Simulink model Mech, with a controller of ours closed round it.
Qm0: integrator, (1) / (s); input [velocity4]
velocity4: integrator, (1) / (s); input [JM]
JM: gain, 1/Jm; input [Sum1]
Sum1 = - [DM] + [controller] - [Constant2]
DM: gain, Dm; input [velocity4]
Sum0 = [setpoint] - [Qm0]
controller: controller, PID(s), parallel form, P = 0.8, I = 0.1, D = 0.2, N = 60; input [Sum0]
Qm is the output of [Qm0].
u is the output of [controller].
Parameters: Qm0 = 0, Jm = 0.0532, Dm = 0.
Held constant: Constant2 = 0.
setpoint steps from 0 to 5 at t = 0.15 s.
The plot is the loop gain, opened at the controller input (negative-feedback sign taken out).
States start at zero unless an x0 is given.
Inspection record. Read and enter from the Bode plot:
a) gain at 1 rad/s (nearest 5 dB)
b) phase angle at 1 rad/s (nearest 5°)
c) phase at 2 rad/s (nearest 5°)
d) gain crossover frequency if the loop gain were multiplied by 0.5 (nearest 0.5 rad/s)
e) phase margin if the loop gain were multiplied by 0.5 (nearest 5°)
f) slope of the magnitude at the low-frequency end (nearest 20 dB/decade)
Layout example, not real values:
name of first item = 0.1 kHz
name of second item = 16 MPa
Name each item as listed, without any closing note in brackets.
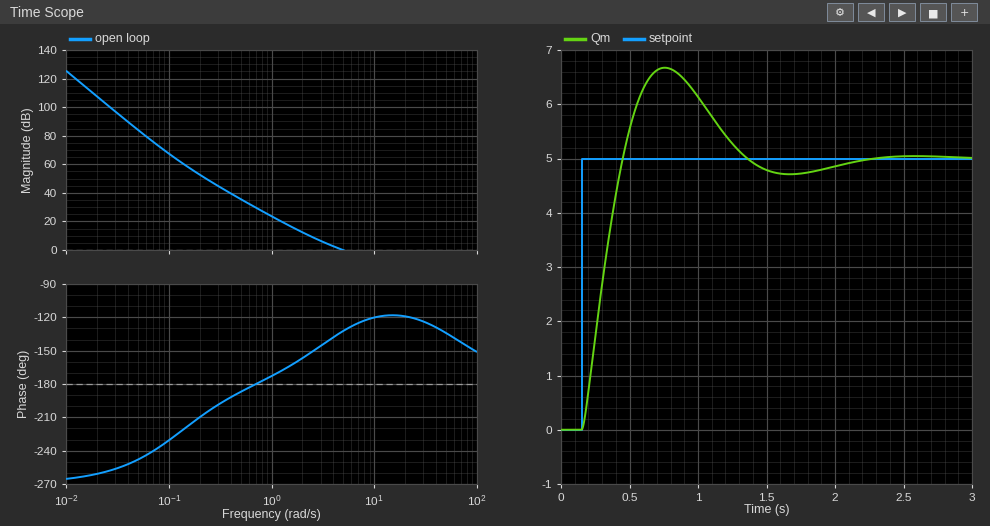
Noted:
gain at 1 rad/s = 25 dB
phase angle at 1 rad/s = -175°
phase at 2 rad/s = -155°
gain crossover frequency if the loop gain were multiplied by 0.5 = 3.0 rad/s
phase margin if the loop gain were multiplied by 0.5 = 35°
slope of the magnitude at the low-frequency end = -60 dB/decade
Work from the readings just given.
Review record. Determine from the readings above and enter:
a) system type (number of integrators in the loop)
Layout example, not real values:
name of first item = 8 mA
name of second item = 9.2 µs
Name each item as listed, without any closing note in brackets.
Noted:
system type = 3
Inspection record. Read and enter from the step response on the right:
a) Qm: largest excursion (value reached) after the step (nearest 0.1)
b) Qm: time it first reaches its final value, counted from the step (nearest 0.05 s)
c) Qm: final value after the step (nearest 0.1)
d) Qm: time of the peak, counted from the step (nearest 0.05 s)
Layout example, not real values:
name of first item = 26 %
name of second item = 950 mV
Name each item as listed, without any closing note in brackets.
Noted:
Qm: largest excursion (value reached) after the step = 6.7
Qm: time it first reaches its final value, counted from the step = 0.30 s
Qm: final value after the step = 5.0
Qm: time of the peak, counted from the step = 0.60 s
